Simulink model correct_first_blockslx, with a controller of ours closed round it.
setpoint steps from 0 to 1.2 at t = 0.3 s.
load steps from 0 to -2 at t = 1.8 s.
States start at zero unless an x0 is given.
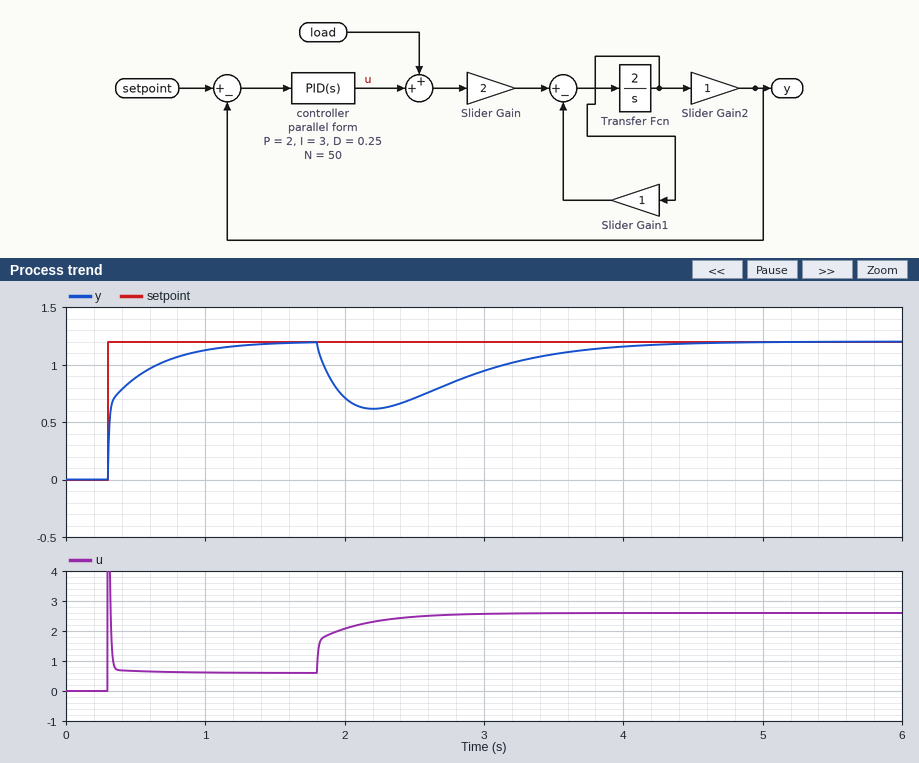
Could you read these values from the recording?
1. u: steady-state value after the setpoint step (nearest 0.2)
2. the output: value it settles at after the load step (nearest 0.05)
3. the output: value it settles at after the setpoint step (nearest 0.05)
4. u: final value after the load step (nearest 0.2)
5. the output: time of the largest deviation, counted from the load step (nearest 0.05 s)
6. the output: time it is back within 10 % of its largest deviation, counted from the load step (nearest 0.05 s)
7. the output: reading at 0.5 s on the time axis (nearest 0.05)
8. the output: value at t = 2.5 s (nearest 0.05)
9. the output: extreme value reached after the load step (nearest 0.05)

0.6
1.20
1.20
2.6
0.40 s
2.05 s
0.90
0.70
0.60
